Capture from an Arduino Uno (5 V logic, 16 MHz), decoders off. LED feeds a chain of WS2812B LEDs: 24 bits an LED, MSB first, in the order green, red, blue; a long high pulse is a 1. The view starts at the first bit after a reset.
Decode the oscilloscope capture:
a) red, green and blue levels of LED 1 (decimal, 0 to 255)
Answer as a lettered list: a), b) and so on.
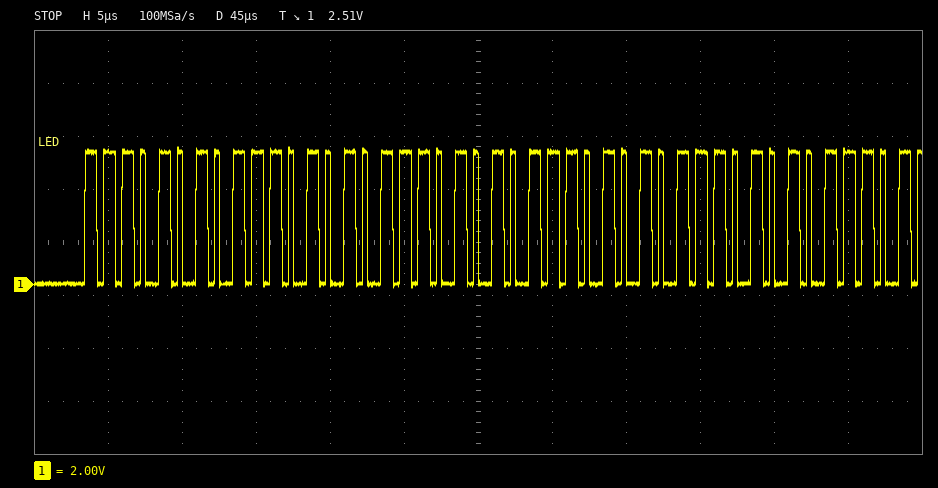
a) 234, 234, 234
